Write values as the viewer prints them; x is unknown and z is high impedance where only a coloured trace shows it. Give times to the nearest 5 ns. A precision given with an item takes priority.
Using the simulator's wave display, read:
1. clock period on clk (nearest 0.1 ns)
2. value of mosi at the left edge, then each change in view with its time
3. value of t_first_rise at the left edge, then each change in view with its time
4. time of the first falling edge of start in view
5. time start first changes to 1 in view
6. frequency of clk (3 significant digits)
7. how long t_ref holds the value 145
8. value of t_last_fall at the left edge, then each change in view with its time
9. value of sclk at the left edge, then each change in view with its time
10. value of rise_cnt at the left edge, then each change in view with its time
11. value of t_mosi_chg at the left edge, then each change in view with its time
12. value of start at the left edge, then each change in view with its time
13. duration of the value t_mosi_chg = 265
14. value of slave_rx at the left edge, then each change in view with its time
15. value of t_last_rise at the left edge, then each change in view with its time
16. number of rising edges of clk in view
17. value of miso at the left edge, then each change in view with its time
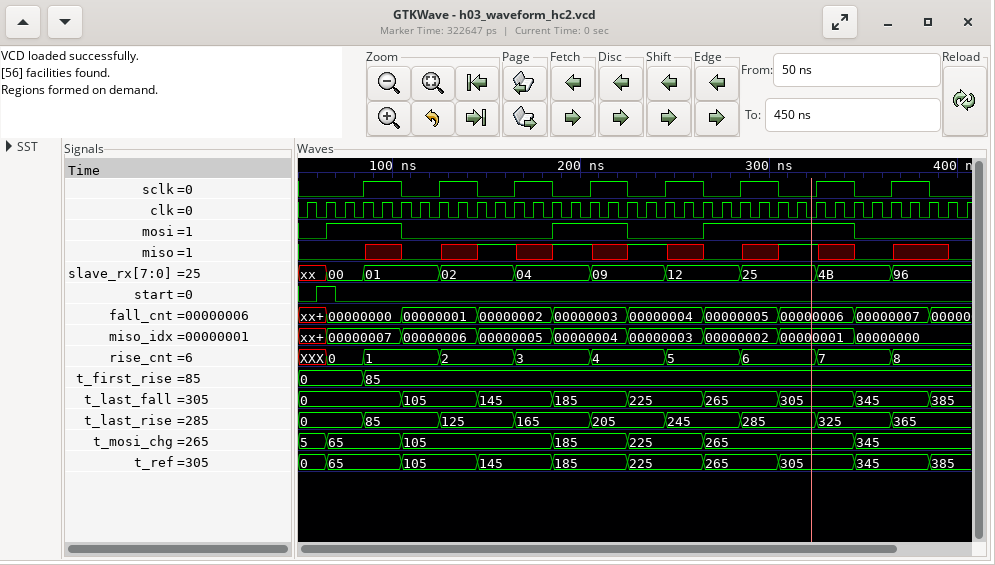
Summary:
10 ns
0, 1 at 65 ns, 0 at 105 ns, 1 at 185 ns, 0 at 225 ns, 1 at 265 ns, 0 at 345 ns
0, 85 at 85 ns
70 ns
60 ns
100 MHz
40 ns
0, 105 at 105 ns, 145 at 145 ns, 185 at 185 ns, 225 at 225 ns, 265 at 265 ns, 305 at 305 ns, 345 at 345 ns, 385 at 385 ns
0, 1 at 85 ns, 0 at 105 ns, 1 at 125 ns, 0 at 145 ns, 1 at 165 ns, 0 at 185 ns, 1 at 205 ns, 0 at 225 ns, 1 at 245 ns, 0 at 265 ns, 1 at 285 ns, 0 at 305 ns, 1 at 325 ns, 0 at 345 ns, 1 at 365 ns, 0 at 385 ns
XXX, 0 at 65 ns, 1 at 85 ns, 2 at 125 ns, 3 at 165 ns, 4 at 205 ns, 5 at 245 ns, 6 at 285 ns, 7 at 325 ns, 8 at 365 ns
5, 65 at 65 ns, 105 at 105 ns, 185 at 185 ns, 225 at 225 ns, 265 at 265 ns, 345 at 345 ns
0, 1 at 60 ns, 0 at 70 ns
80 ns
xx, 00 at 65 ns, 01 at 85 ns, 02 at 125 ns, 04 at 165 ns, 09 at 205 ns, 12 at 245 ns, 25 at 285 ns, 4B at 325 ns, 96 at 365 ns
0, 85 at 85 ns, 125 at 125 ns, 165 at 165 ns, 205 at 205 ns, 245 at 245 ns, 285 at 285 ns, 325 at 325 ns, 365 at 365 ns
36
0, x at 85 ns, 0 at 105 ns, x at 125 ns, 1 at 145 ns, x at 165 ns, 1 at 185 ns, x at 205 ns, 1 at 225 ns, x at 245 ns, 0 at 265 ns, x at 285 ns, 1 at 305 ns, x at 325 ns, 0 at 345 ns, x at 365 ns, 0 at 395 ns
